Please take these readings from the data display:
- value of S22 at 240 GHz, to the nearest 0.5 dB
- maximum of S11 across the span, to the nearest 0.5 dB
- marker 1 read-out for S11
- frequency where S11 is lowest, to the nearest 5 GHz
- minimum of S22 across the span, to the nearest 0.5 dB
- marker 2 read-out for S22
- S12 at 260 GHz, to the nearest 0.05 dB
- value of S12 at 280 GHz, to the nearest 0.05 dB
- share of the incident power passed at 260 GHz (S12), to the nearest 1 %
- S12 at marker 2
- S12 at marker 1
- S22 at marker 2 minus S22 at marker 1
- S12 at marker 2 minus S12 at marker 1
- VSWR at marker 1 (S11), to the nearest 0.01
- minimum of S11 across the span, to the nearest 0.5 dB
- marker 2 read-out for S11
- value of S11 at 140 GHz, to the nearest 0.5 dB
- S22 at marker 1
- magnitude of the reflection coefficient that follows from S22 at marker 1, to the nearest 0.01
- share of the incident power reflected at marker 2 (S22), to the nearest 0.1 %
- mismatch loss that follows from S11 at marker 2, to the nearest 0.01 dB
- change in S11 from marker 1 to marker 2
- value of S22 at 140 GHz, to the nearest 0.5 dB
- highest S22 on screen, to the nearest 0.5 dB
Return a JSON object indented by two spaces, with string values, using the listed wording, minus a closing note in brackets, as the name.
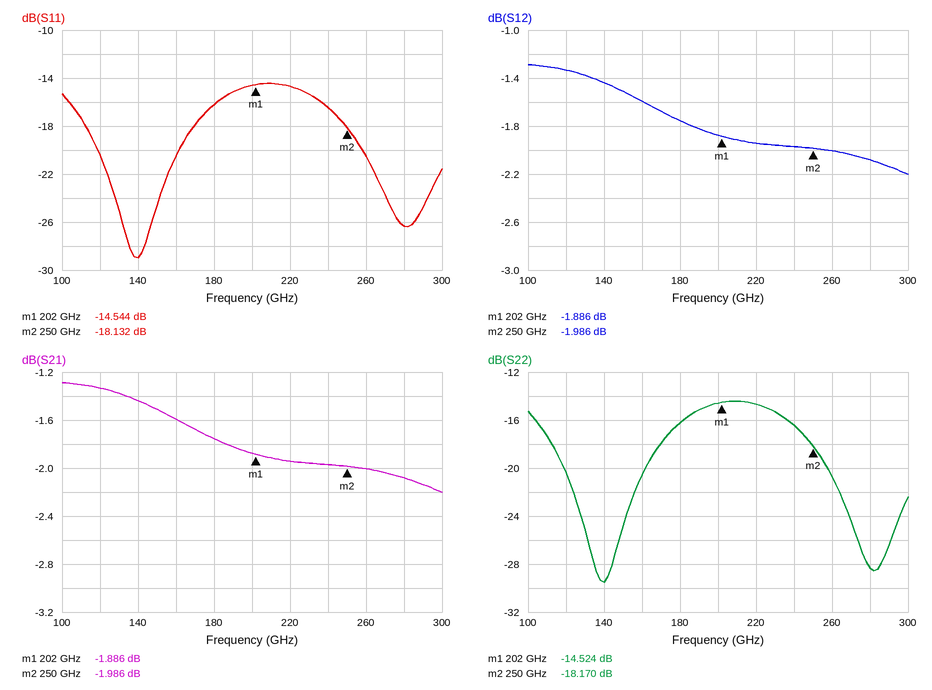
{
  "value of S22 at 240 GHz, to the nearest 0.5 dB": "-16.5 dB",
  "maximum of S11 across the span, to the nearest 0.5 dB": "-14.5 dB",
  "marker 1 read-out for S11": "-14.544 dB",
  "frequency where S11 is lowest, to the nearest 5 GHz": "140 GHz",
  "minimum of S22 across the span, to the nearest 0.5 dB": "-29.5 dB",
  "marker 2 read-out for S22": "-18.170 dB",
  "S12 at 260 GHz, to the nearest 0.05 dB": "-2.00 dB",
  "value of S12 at 280 GHz, to the nearest 0.05 dB": "-2.10 dB",
  "share of the incident power passed at 260 GHz (S12), to the nearest 1 %": "63 %",
  "S12 at marker 2": "-1.986 dB",
  "S12 at marker 1": "-1.886 dB",
  "S22 at marker 2 minus S22 at marker 1": "-3.646 dB",
  "S12 at marker 2 minus S12 at marker 1": "-0.100 dB",
  "VSWR at marker 1 (S11), to the nearest 0.01": "1.46",
  "minimum of S11 across the span, to the nearest 0.5 dB": "-29.0 dB",
  "marker 2 read-out for S11": "-18.132 dB",
  "value of S11 at 140 GHz, to the nearest 0.5 dB": "-29.0 dB",
  "S22 at marker 1": "-14.524 dB",
  "magnitude of the reflection coefficient that follows from S22 at marker 1, to the nearest 0.01": "0.19",
  "share of the incident power reflected at marker 2 (S22), to the nearest 0.1 %": "1.5 %",
  "mismatch loss that follows from S11 at marker 2, to the nearest 0.01 dB": "0.07 dB",
  "change in S11 from marker 1 to marker 2": "-3.588 dB",
  "value of S22 at 140 GHz, to the nearest 0.5 dB": "-29.5 dB",
  "highest S22 on screen, to the nearest 0.5 dB": "-14.5 dB"
}
